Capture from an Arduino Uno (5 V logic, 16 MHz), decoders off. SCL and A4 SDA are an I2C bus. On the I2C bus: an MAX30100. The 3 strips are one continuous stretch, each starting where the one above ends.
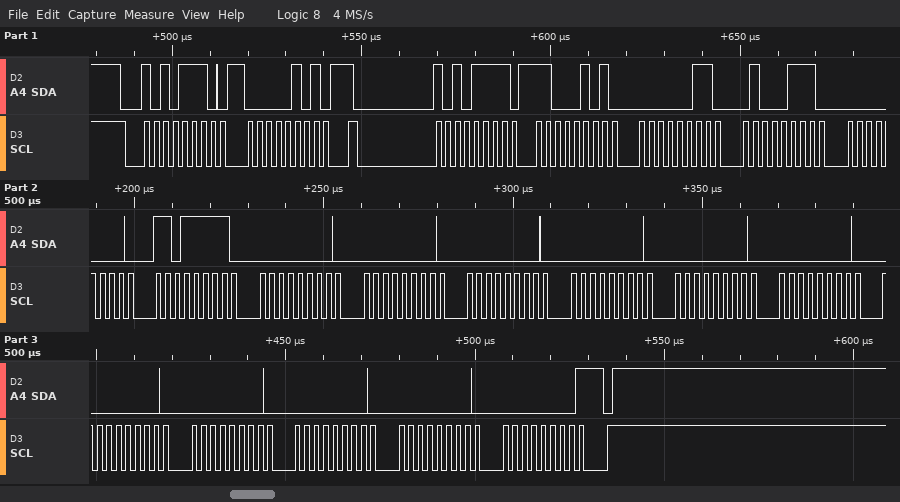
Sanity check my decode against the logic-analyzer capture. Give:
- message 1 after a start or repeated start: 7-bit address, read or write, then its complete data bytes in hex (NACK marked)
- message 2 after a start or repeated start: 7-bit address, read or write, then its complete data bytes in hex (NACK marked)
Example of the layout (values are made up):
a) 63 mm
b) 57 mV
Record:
a) 0x57 write: 05
b) 0x57 read: C5 03 47 00 DF 00 00 00 00 00 00 00 00 00 00 00 NACK
